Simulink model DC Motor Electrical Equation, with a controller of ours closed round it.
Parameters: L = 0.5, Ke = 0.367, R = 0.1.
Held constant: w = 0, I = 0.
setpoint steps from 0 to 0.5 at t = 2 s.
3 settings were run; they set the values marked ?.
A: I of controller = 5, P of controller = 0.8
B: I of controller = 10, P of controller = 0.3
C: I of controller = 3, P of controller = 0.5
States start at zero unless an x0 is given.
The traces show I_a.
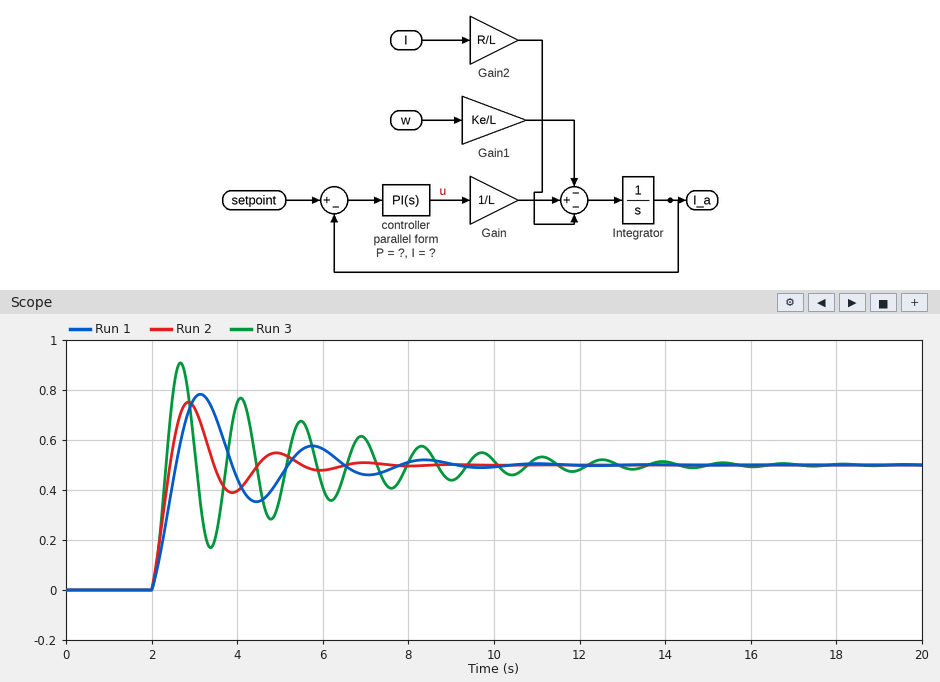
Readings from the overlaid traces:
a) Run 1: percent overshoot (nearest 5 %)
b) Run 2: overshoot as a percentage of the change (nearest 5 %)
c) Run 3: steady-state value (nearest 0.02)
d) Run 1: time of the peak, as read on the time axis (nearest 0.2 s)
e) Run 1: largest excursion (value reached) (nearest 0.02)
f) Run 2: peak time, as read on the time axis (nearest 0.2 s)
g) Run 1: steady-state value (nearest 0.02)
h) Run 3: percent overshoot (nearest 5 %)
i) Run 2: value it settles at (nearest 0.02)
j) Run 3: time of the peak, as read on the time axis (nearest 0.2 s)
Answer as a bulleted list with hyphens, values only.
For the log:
- 55 %
- 50 %
- 0.50
- 3.2 s
- 0.78
- 2.8 s
- 0.50
- 80 %
- 0.50
- 2.6 s
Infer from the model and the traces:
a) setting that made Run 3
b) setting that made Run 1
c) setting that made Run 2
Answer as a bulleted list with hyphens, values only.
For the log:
- B
- C
- A
